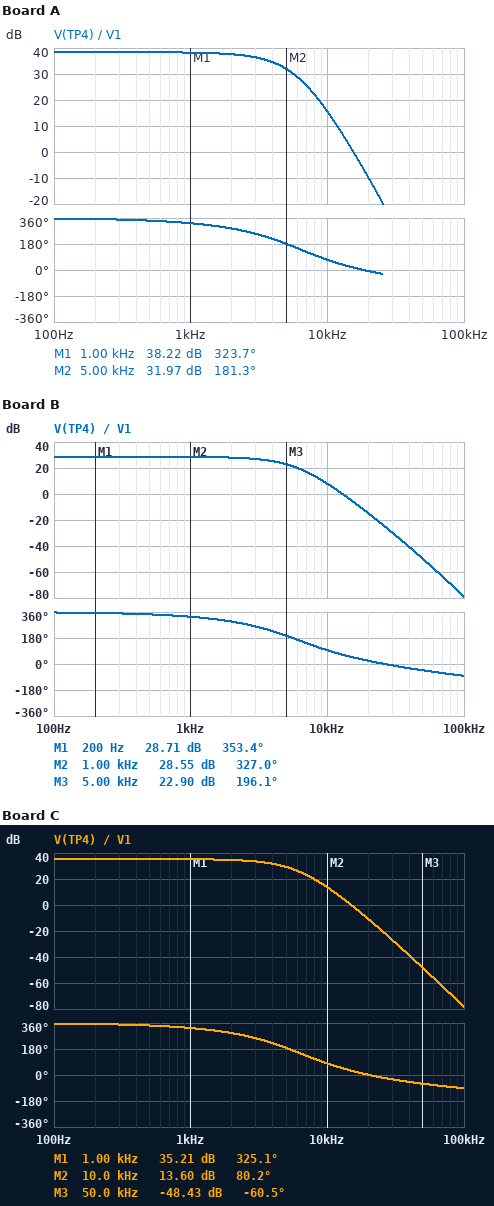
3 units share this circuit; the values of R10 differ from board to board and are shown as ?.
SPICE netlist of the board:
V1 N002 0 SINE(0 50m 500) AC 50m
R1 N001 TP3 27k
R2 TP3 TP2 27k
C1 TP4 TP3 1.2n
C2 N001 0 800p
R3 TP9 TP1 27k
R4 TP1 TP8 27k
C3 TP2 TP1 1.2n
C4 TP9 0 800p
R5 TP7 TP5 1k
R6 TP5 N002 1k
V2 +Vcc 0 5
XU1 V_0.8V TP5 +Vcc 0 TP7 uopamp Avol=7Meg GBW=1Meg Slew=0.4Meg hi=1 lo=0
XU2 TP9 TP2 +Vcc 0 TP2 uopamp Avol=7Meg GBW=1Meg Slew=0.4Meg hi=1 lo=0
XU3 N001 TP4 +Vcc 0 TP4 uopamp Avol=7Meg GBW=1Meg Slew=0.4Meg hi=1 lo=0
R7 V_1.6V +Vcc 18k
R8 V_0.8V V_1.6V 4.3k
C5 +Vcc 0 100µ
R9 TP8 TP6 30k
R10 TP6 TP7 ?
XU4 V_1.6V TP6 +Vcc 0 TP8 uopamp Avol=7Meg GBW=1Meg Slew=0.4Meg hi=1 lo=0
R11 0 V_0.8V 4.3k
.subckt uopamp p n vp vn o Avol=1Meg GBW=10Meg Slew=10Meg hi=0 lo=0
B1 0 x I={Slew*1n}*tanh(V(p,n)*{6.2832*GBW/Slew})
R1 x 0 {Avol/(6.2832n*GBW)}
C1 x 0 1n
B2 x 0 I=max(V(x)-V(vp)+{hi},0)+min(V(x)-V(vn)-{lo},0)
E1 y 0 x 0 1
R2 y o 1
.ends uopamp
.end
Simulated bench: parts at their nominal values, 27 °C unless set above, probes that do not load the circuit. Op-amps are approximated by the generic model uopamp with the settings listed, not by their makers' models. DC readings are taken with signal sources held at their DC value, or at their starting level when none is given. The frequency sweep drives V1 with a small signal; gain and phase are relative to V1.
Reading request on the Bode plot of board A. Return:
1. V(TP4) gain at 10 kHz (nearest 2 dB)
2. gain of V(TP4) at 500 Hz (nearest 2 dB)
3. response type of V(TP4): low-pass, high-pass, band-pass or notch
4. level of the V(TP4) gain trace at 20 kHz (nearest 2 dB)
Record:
16 dB
38 dB
low-pass
-10 dB
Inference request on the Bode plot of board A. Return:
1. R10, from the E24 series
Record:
360 Ω
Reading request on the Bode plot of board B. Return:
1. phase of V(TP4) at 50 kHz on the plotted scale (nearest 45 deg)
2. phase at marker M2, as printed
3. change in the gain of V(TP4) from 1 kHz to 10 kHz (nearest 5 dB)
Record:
-45 deg
327.0 deg
-20 dB
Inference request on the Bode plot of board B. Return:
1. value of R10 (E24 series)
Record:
1.1 kΩ
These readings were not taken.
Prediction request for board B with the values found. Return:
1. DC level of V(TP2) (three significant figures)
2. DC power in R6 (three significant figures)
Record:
1.62 V
653 µW
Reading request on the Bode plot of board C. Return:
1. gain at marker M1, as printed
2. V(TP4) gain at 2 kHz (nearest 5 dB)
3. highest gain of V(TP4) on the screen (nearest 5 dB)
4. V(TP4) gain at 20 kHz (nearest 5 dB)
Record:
35.21 dB
35 dB
35 dB
-10 dB
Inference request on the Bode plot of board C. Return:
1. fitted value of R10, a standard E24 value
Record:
510 Ω
